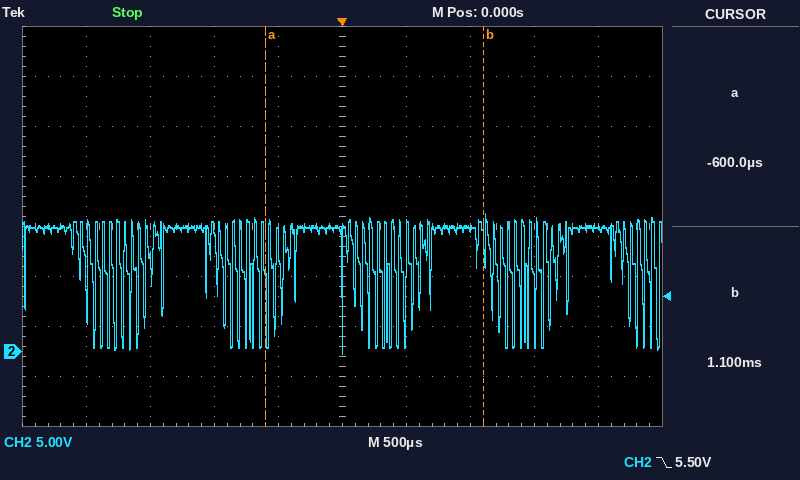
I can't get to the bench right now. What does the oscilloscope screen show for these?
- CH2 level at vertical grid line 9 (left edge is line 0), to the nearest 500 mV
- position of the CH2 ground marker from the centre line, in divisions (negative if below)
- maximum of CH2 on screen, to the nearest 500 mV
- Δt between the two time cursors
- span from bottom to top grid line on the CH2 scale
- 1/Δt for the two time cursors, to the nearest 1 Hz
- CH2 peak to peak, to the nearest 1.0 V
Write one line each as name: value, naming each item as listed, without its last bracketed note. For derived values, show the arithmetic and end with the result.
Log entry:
CH2 level at vertical grid line 9 (left edge is line 0), to the nearest 500 mV: 12.5 V
position of the CH2 ground marker from the centre line, in divisions: -2.5 div
maximum of CH2 on screen, to the nearest 500 mV: 14.0 V
Δt between the two time cursors: 1.1 ms − (-600 µs) = 1.70 ms
span from bottom to top grid line on the CH2 scale: 40 V
1/Δt for the two time cursors, to the nearest 1 Hz: 1 / 1.70 ms ≈ 588 Hz
CH2 peak to peak, to the nearest 1.0 V: 14.0 V
